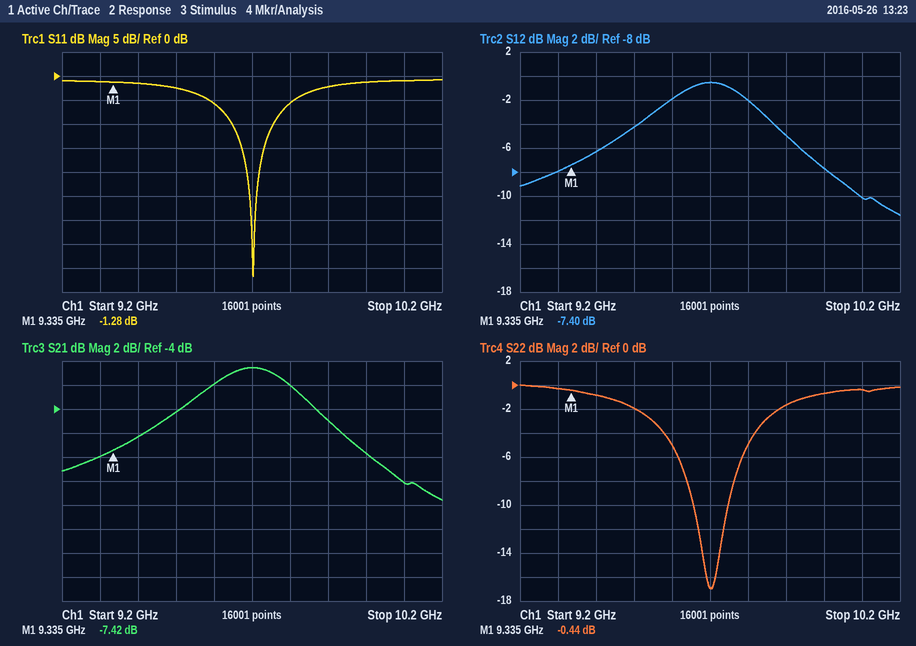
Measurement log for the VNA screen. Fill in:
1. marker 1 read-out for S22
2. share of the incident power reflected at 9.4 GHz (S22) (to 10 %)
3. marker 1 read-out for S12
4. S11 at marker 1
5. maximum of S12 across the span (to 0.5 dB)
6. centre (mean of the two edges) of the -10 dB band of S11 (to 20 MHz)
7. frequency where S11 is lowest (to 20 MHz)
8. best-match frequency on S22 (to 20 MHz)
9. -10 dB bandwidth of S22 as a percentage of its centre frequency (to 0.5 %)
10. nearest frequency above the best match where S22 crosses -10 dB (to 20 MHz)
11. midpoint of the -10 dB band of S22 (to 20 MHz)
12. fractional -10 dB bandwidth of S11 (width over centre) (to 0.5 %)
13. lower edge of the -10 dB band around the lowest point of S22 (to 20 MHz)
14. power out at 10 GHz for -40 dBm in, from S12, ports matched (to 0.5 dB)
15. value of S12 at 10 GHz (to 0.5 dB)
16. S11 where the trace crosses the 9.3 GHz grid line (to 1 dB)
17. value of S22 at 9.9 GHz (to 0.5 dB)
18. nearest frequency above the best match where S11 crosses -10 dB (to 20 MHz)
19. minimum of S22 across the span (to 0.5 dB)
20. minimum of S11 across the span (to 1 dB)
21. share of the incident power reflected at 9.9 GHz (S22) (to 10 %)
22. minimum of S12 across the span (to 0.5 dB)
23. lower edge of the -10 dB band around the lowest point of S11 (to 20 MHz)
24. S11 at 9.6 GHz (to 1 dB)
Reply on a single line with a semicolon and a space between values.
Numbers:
-0.44 dB; 80 %; -7.40 dB; -1.28 dB; -0.5 dB; 9.70 GHz; 9.70 GHz; 9.70 GHz; 1.0 %; 9.74 GHz; 9.70 GHz; 1.0 %; 9.66 GHz; -47.5 dBm; -7.5 dB; -1 dB; -1.5 dB; 9.76 GHz; -17.0 dB; -42 dB; 70 %; -11.5 dB; 9.64 GHz; -6 dB
